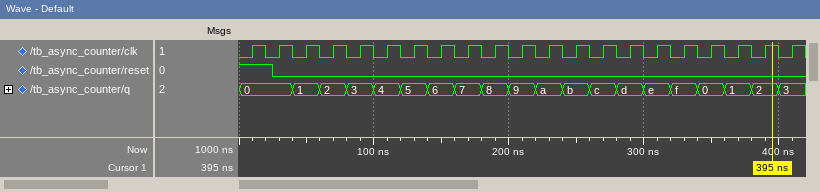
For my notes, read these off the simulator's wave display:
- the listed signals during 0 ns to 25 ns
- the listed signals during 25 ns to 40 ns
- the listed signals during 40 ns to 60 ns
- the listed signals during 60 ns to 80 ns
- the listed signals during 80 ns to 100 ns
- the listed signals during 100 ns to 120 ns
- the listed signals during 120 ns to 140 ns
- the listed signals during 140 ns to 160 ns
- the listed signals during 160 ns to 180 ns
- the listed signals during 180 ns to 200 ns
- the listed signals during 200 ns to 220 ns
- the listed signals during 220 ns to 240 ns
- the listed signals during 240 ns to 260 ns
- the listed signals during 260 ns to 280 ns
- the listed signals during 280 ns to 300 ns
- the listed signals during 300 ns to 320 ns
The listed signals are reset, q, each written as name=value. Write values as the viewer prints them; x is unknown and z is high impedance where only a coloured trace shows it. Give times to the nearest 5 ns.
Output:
reset=1, q=0
reset=0, q=0
reset=0, q=1
reset=0, q=2
reset=0, q=3
reset=0, q=4
reset=0, q=5
reset=0, q=6
reset=0, q=7
reset=0, q=8
reset=0, q=9
reset=0, q=a
reset=0, q=b
reset=0, q=c
reset=0, q=d
reset=0, q=e
